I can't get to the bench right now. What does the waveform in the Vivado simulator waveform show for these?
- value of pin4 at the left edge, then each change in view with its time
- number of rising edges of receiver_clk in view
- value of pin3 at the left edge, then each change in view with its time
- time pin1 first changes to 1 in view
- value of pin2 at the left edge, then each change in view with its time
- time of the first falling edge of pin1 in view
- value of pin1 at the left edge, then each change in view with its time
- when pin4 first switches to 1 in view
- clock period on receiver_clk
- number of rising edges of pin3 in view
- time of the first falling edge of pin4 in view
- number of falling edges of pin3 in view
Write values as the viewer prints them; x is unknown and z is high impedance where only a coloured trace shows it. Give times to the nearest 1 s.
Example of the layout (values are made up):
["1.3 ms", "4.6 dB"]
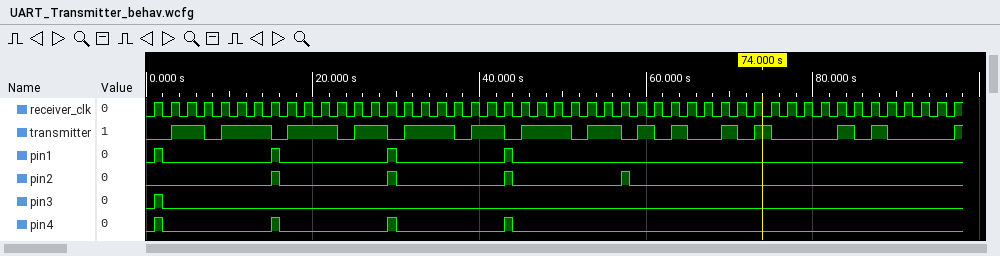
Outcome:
["0, 1 at 1 s, 0 at 2 s, 1 at 15 s, 0 at 16 s, 1 at 29 s, 0 at 30 s, 1 at 43 s, 0 at 44 s", "49", "0, 1 at 1 s, 0 at 2 s", "1 s", "0, 1 at 15 s, 0 at 16 s, 1 at 29 s, 0 at 30 s, 1 at 43 s, 0 at 44 s, 1 at 57 s, 0 at 58 s", "2 s", "0, 1 at 1 s, 0 at 2 s, 1 at 15 s, 0 at 16 s, 1 at 29 s, 0 at 30 s, 1 at 43 s, 0 at 44 s", "1 s", "2 s", "1", "2 s", "1"]
